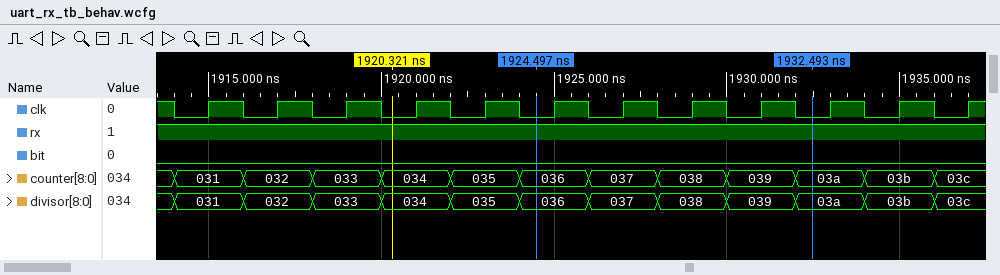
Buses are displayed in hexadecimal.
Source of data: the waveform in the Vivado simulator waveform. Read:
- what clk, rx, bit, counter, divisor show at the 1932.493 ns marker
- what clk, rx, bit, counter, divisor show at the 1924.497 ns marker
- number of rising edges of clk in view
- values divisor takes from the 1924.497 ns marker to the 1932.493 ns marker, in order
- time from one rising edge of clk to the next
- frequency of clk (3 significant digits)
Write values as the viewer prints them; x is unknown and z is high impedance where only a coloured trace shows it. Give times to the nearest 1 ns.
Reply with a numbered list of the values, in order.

1. clk=0, rx=1, bit=0, counter=03a, divisor=03a
2. clk=0, rx=1, bit=0, counter=036, divisor=036
3. 12
4. 036, 037, 038, 039, 03a
5. 2 ns
6. 500 MHz
